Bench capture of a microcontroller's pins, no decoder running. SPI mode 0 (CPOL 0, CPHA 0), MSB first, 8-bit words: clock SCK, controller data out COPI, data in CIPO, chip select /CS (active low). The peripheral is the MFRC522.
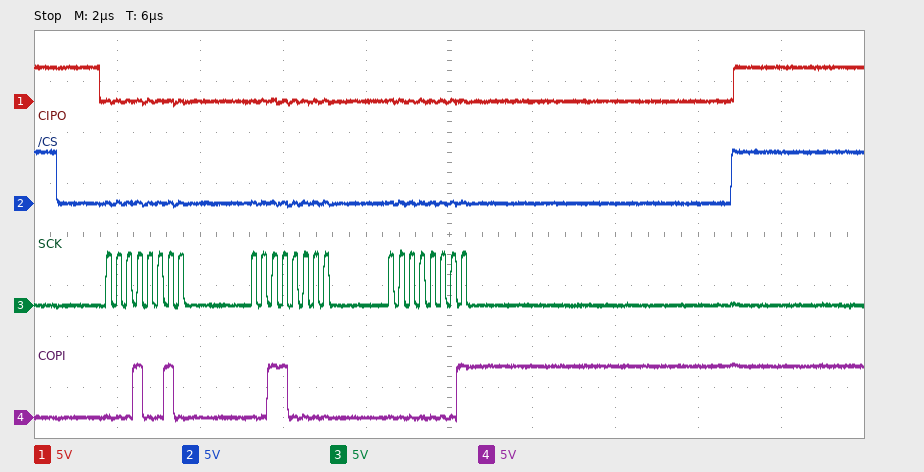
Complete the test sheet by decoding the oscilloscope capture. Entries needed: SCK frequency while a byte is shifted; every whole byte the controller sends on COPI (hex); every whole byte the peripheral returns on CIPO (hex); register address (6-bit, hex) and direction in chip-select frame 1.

4 MHz
12 30 01
00 00 00
0x09 write
